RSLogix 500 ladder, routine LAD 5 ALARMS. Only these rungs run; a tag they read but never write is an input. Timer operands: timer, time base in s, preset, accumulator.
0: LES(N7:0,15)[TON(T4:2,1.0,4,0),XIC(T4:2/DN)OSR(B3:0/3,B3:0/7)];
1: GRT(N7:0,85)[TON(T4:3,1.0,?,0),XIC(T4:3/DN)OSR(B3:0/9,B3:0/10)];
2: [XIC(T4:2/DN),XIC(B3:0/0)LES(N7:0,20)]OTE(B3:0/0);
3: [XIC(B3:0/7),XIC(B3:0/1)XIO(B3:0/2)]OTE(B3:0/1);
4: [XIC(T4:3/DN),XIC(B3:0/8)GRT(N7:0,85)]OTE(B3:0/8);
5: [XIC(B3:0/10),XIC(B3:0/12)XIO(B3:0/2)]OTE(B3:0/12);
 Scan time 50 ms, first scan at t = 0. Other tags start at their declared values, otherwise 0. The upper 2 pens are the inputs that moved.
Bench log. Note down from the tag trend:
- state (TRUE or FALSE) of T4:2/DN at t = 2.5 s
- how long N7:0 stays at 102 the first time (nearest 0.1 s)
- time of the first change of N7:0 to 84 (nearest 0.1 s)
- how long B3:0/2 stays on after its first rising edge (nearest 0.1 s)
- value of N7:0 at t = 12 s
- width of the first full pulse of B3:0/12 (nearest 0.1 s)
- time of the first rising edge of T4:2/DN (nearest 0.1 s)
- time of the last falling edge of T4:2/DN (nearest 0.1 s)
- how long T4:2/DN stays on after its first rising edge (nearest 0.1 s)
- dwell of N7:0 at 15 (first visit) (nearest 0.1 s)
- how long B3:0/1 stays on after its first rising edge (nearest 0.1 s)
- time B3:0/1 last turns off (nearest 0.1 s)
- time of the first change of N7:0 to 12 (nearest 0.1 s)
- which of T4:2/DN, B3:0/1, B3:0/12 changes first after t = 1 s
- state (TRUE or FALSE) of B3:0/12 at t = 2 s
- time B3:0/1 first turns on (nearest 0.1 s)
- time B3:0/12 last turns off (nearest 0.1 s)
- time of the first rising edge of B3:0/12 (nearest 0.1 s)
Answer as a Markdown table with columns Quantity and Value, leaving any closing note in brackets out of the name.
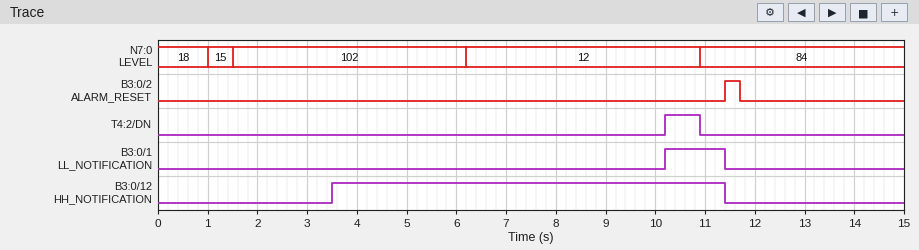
| Quantity | Value |
|---|---|
| state (TRUE or FALSE) of T4:2/DN at t = 2.5 s | FALSE |
| how long N7:0 stays at 102 the first time | 4.7 s |
| time of the first change of N7:0 to 84 | 10.9 s |
| how long B3:0/2 stays on after its first rising edge | 0.3 s |
| value of N7:0 at t = 12 s | 84 |
| width of the first full pulse of B3:0/12 | 7.9 s |
| time of the first rising edge of T4:2/DN | 10.2 s |
| time of the last falling edge of T4:2/DN | 10.9 s |
| how long T4:2/DN stays on after its first rising edge | 0.7 s |
| dwell of N7:0 at 15 (first visit) | 0.5 s |
| how long B3:0/1 stays on after its first rising edge | 1.2 s |
| time B3:0/1 last turns off | 11.4 s |
| time of the first change of N7:0 to 12 | 6.2 s |
| which of T4:2/DN, B3:0/1, B3:0/12 changes first after t = 1 s | B3:0/12 |
| state (TRUE or FALSE) of B3:0/12 at t = 2 s | FALSE |
| time B3:0/1 first turns on | 10.2 s |
| time B3:0/12 last turns off | 11.4 s |
| time of the first rising edge of B3:0/12 | 3.5 s |
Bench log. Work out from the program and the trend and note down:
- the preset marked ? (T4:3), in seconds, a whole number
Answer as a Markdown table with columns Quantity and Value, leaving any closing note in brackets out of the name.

| Quantity | Value |
|---|---|
| the preset marked ? (T4:3), in seconds, a whole number | 2 s |
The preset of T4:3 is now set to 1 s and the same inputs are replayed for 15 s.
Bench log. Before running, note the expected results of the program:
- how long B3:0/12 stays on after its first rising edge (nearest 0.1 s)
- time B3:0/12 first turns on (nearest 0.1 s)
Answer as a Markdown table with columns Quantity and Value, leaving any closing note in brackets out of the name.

| Quantity | Value |
|---|---|
| how long B3:0/12 stays on after its first rising edge | 8.9 s |
| time B3:0/12 first turns on | 2.5 s |
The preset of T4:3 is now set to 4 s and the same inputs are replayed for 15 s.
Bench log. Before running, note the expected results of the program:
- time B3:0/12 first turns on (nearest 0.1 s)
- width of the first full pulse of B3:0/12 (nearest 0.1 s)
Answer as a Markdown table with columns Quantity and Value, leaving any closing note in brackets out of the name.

| Quantity | Value |
|---|---|
| time B3:0/12 first turns on | 5.5 s |
| width of the first full pulse of B3:0/12 | 5.9 s |
